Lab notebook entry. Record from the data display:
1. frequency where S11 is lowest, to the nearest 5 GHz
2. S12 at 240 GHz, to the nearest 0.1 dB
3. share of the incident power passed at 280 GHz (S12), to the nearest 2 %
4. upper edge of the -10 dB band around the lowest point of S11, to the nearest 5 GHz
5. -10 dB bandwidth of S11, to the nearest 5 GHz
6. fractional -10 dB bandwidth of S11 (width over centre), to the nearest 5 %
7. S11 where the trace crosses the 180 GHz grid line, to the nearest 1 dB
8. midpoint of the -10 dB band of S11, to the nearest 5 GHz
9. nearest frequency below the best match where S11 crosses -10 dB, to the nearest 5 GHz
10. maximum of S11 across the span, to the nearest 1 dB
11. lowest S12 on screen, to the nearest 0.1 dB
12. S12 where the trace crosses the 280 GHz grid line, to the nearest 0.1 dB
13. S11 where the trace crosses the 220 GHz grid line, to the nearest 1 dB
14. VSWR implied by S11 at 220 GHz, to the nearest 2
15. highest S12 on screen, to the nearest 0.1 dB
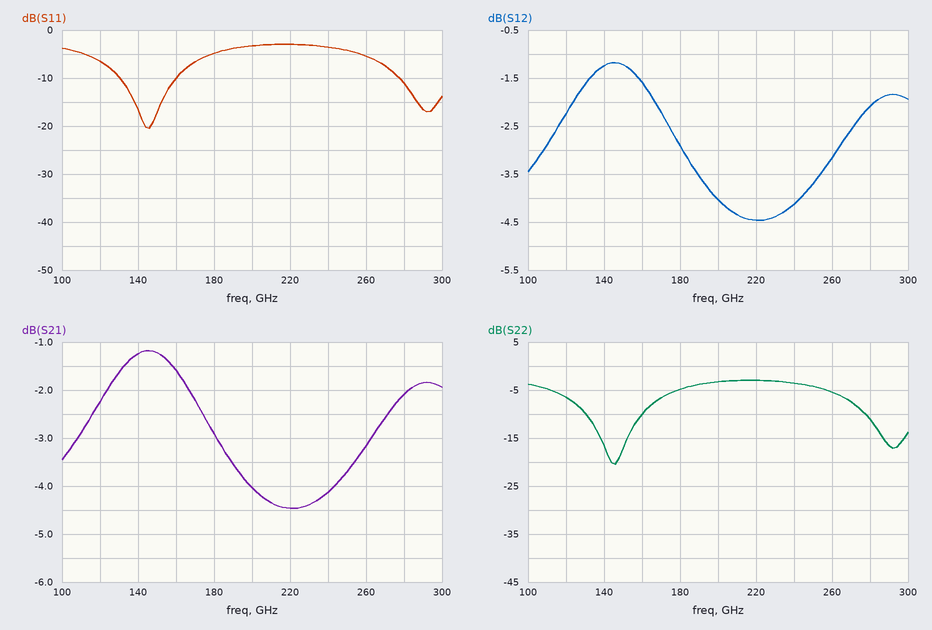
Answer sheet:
145 GHz
-4.1 dB
62 %
160 GHz
30 GHz
20 %
-5 dB
145 GHz
130 GHz
-3 dB
-4.5 dB
-2.1 dB
-3 dB
6
-1.2 dB
